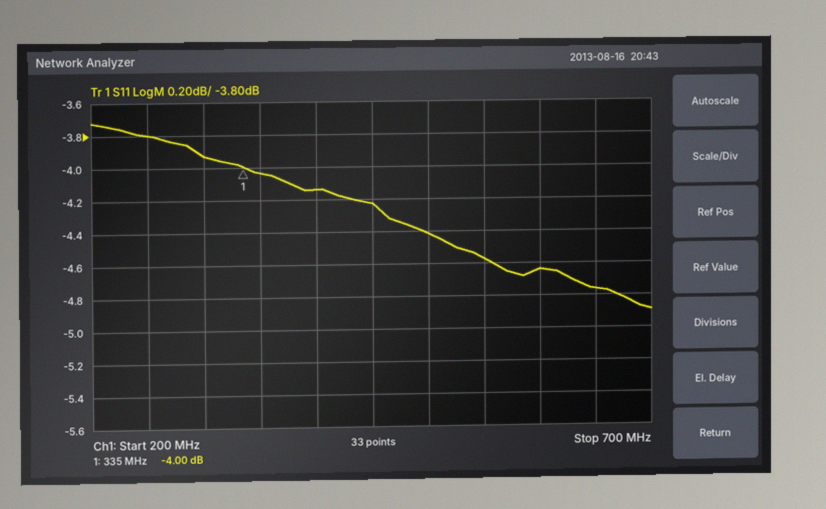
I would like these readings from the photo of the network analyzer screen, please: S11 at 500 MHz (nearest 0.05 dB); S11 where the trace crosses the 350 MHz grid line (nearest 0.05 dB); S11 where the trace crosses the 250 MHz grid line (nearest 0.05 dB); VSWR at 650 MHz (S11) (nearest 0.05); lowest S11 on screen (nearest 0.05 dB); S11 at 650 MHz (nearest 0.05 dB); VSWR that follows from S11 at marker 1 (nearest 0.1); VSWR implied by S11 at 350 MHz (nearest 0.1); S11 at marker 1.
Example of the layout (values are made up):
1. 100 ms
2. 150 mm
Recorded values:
1. -4.40 dB
2. -4.05 dB
3. -3.80 dB
4. 3.75
5. -4.90 dB
6. -4.75 dB
7. 4.4
8. 4.4
9. -4.00 dB
